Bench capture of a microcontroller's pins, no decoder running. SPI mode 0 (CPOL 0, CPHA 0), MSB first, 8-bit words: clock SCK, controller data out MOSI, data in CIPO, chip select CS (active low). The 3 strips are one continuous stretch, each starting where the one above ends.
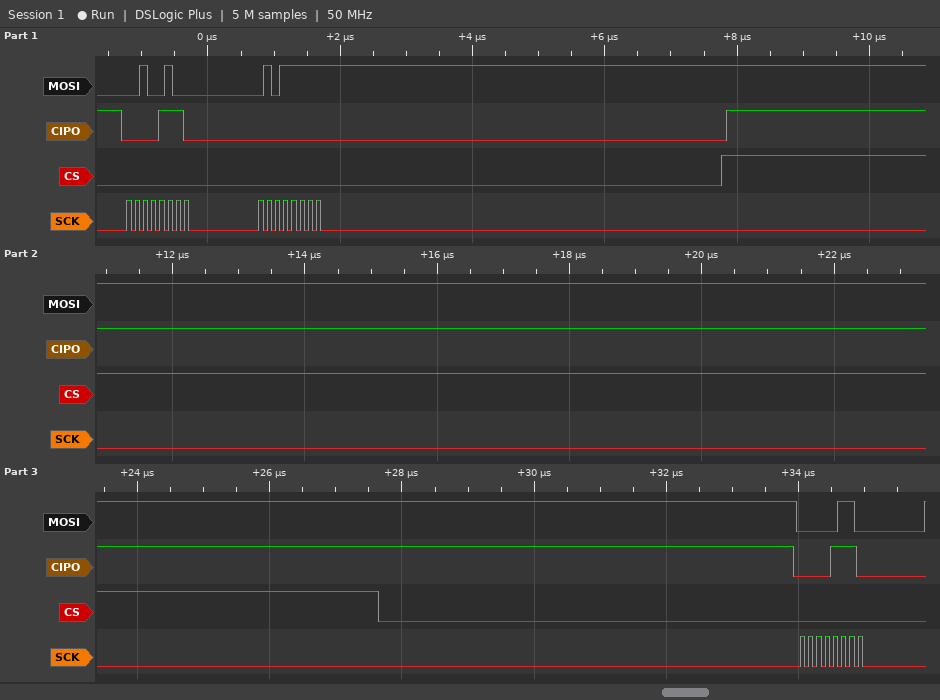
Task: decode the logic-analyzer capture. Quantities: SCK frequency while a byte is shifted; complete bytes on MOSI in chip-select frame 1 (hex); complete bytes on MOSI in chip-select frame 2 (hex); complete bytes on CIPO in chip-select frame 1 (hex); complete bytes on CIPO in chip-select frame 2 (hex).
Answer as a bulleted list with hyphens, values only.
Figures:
- 8 MHz
- 24 5F
- 06
- 0E 00
- 0E
